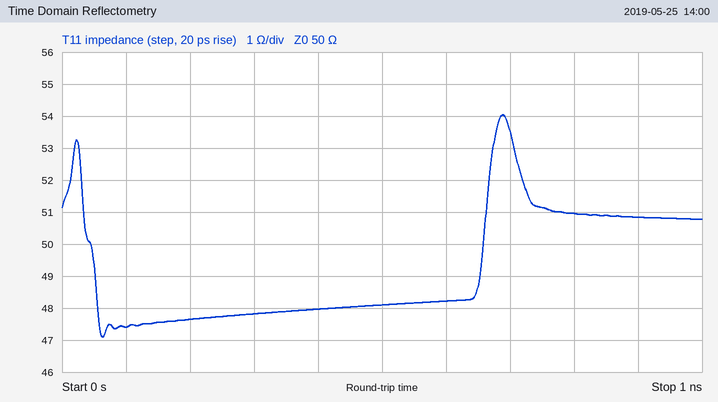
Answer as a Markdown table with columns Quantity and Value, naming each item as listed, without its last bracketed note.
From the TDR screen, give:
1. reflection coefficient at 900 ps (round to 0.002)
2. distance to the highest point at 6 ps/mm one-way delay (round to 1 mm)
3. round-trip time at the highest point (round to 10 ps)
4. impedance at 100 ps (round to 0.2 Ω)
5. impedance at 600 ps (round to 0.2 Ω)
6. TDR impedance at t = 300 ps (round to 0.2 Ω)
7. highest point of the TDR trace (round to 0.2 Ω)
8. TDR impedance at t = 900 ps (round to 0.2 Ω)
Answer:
| Quantity | Value |
|---|---|
| reflection coefficient at 900 ps | +0.008 |
| distance to the highest point at 6 ps/mm one-way delay | 57 mm |
| round-trip time at the highest point | 690 ps |
| impedance at 100 ps | 47.4 Ω |
| impedance at 600 ps | 48.2 Ω |
| TDR impedance at t = 300 ps | 47.8 Ω |
| highest point of the TDR trace | 54.0 Ω |
| TDR impedance at t = 900 ps | 50.8 Ω |
